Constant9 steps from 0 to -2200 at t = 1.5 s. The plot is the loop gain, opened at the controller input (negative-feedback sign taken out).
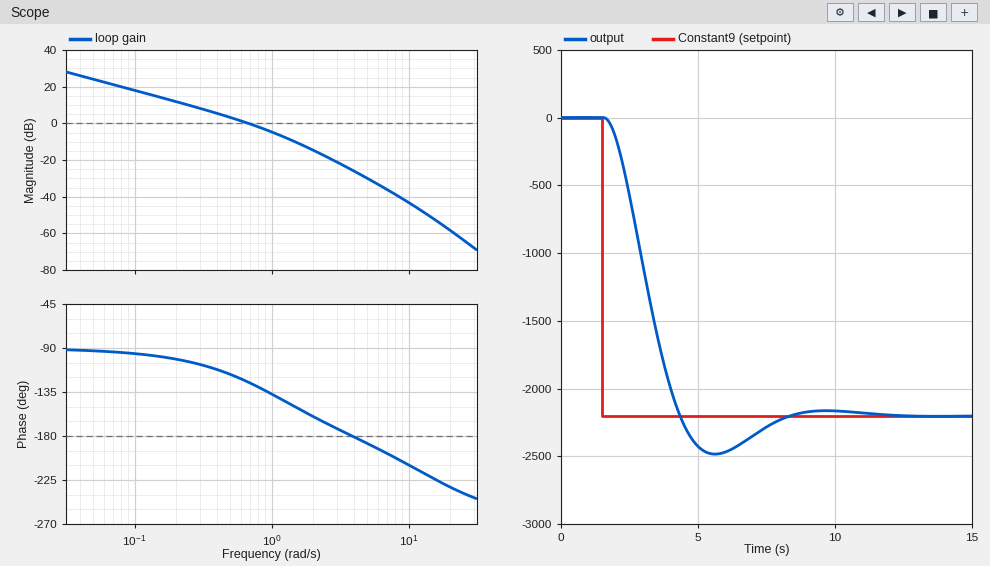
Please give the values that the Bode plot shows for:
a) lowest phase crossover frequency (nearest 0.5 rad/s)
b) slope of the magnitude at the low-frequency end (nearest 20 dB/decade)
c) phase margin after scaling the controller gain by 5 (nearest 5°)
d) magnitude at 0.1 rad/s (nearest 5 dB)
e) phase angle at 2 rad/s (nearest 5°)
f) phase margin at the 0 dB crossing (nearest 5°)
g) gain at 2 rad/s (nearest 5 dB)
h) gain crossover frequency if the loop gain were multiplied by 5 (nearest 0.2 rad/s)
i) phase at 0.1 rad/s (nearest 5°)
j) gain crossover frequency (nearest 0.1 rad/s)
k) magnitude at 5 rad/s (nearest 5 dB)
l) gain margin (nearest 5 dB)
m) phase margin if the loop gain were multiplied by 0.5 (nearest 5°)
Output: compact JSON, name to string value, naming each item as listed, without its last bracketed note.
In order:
{"lowest phase crossover frequency": "4.0 rad/s", "slope of the magnitude at the low-frequency end": "-20 dB/decade", "phase margin after scaling the controller gain by 5": "20°", "magnitude at 0.1 rad/s": "20 dB", "phase angle at 2 rad/s": "-160°", "phase margin at the 0 dB crossing": "55°", "gain at 2 rad/s": "-15 dB", "gain crossover frequency if the loop gain were multiplied by 5": "2.0 rad/s", "phase at 0.1 rad/s": "-95°", "gain crossover frequency": "0.7 rad/s", "magnitude at 5 rad/s": "-30 dB", "gain margin": "25 dB", "phase margin if the loop gain were multiplied by 0.5": "70°"}
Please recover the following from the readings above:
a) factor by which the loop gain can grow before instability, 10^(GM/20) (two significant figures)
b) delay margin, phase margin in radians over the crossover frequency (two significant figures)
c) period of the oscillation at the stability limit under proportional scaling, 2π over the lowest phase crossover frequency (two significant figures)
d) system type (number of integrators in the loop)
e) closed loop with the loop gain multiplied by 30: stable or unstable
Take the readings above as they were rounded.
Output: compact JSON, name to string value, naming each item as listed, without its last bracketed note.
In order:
{"factor by which the loop gain can grow before instability, 10^(GM/20)": "18", "delay margin, phase margin in radians over the crossover frequency": "1.4 s", "period of the oscillation at the stability limit under proportional scaling, 2π over the lowest phase crossover frequency": "1.6 s", "system type": "1", "closed loop with the loop gain multiplied by 30: stable or unstable": "unstable"}
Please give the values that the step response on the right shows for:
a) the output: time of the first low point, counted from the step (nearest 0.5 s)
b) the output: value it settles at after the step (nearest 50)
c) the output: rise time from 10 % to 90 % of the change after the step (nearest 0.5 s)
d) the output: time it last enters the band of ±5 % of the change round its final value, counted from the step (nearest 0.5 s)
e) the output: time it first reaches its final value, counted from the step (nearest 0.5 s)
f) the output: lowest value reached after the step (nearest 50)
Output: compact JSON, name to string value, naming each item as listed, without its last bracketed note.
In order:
{"the output: time of the first low point, counted from the step": "4.0 s", "the output: value it settles at after the step": "-2200", "the output: rise time from 10 % to 90 % of the change after the step": "2.0 s", "the output: time it last enters the band of ±5 % of the change round its final value, counted from the step": "6.0 s", "the output: time it first reaches its final value, counted from the step": "3.0 s", "the output: lowest value reached after the step": "-2500"}
